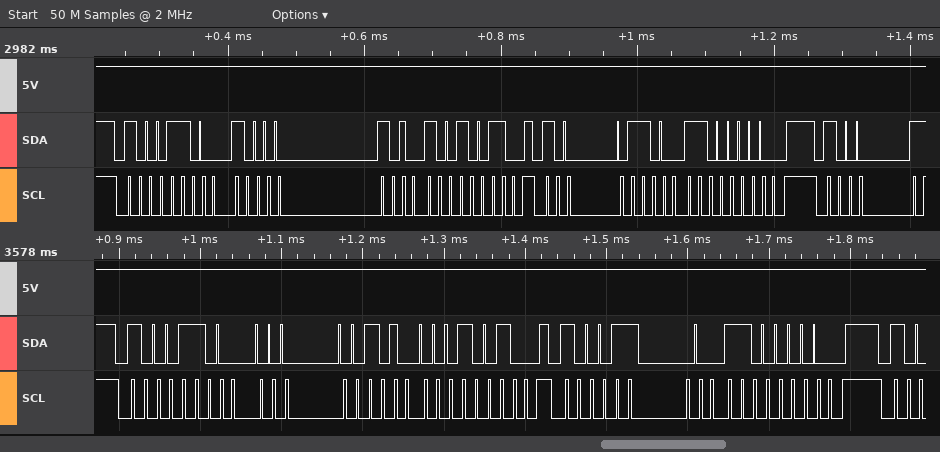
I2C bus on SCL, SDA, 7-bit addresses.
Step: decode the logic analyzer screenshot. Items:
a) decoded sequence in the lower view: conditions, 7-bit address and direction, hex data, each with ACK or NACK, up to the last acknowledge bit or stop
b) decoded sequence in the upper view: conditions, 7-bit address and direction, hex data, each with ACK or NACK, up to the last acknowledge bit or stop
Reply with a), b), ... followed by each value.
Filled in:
a) start, address 46 write ACK, 05 ACK, 12 ACK, stop, start, address 46 write ACK, C0 ACK, stop
b) start, address 46 write ACK, 85 ACK, 93 ACK, stop, start, address 46 write ACK, C0 ACK, stop
